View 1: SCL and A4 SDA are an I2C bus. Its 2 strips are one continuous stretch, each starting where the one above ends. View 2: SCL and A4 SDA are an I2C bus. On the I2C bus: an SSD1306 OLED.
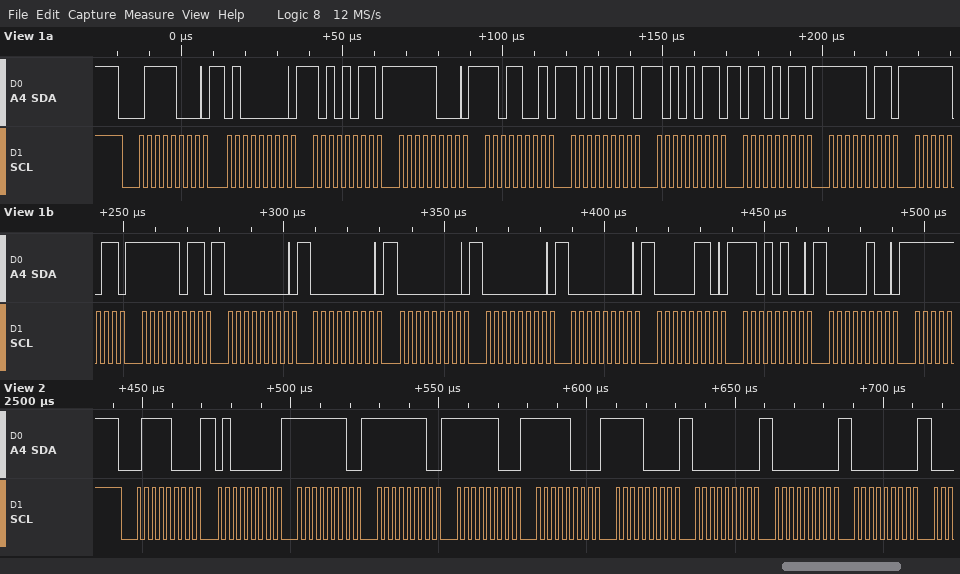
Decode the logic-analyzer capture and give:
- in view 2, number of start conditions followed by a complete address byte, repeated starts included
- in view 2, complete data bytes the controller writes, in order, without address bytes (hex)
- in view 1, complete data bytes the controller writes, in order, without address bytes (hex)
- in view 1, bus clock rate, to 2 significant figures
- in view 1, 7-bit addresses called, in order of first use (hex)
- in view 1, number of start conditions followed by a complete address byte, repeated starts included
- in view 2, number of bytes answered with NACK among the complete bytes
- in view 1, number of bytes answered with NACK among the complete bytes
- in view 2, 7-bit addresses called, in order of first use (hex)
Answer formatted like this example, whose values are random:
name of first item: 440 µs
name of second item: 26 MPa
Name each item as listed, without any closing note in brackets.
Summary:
in view 2, number of start conditions followed by a complete address byte, repeated starts included: 1
in view 2, complete data bytes the controller writes, in order, without address bytes: 40 FE FE FC F8 F0 00 00 00
in view 1, complete data bytes the controller writes, in order, without address bytes: 40 AB F8 D9 AB AB 6B FB FB FB 00 00 00 00 00 06 D4 04
in view 1, bus clock rate, to 2 significant figures: 400 kHz
in view 1, 7-bit addresses called, in order of first use: 0x3C
in view 1, number of start conditions followed by a complete address byte, repeated starts included: 1
in view 2, number of bytes answered with NACK among the complete bytes: 0
in view 1, number of bytes answered with NACK among the complete bytes: 0
in view 2, 7-bit addresses called, in order of first use: 0x3C
